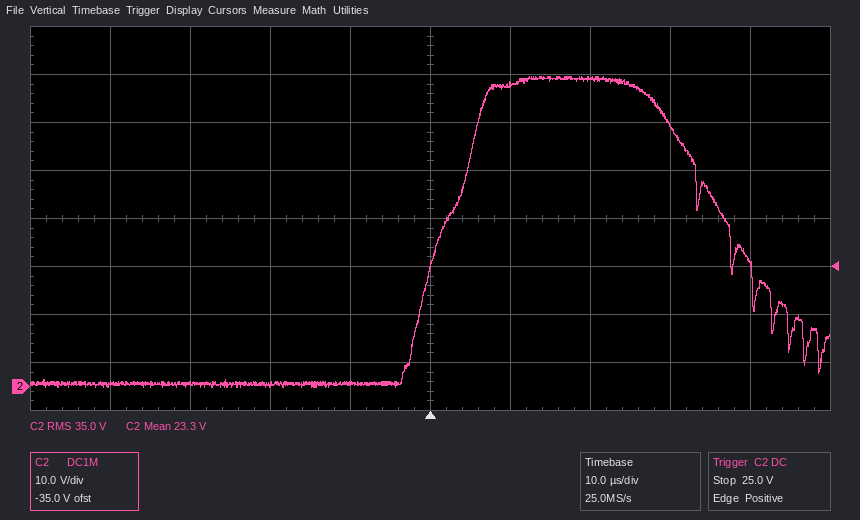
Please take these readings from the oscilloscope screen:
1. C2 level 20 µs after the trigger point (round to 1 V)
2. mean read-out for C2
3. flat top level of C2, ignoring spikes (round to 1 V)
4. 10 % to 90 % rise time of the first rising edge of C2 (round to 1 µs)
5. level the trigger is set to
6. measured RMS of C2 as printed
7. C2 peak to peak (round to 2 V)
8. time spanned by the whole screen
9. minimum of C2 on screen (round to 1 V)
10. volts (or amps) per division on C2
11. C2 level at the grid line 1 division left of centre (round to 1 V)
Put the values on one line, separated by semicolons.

64 V; 23.3 V; 64 V; 9 µs; 25.0 V; 35.0 V; 64 V; 100 µs; 0 V; 10 V; 1 V
